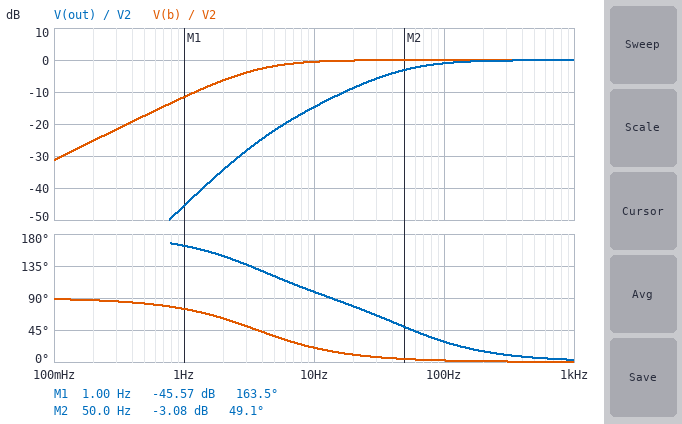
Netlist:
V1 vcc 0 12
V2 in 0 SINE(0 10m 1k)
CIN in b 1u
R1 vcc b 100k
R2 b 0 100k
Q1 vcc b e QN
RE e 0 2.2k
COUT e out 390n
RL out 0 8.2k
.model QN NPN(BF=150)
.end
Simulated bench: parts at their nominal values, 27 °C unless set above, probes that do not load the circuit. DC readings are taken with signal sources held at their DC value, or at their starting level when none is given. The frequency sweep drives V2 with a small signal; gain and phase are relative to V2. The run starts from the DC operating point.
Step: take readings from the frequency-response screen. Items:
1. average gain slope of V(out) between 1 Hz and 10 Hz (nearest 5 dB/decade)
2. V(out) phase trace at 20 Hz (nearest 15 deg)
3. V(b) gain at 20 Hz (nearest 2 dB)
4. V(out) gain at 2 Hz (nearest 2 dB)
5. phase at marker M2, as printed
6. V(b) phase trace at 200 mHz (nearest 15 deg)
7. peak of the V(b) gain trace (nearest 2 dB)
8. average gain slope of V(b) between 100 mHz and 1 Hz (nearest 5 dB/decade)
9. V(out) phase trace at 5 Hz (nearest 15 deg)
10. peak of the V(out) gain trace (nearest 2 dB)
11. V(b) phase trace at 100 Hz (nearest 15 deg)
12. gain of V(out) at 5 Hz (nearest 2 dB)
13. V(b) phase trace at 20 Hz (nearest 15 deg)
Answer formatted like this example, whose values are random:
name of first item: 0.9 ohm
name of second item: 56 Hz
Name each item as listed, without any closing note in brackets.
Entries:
average gain slope of V(out) between 1 Hz and 10 Hz: 30 dB/decade
V(out) phase trace at 20 Hz: 75 deg
V(b) gain at 20 Hz: 0 dB
V(out) gain at 2 Hz: -34 dB
phase at marker M2, as printed: 49.1 deg
V(b) phase trace at 200 mHz: 90 deg
peak of the V(b) gain trace: 0 dB
average gain slope of V(b) between 100 mHz and 1 Hz: 20 dB/decade
V(out) phase trace at 5 Hz: 120 deg
peak of the V(out) gain trace: 0 dB
V(b) phase trace at 100 Hz: 0 deg
gain of V(out) at 5 Hz: -22 dB
V(b) phase trace at 20 Hz: 15 deg
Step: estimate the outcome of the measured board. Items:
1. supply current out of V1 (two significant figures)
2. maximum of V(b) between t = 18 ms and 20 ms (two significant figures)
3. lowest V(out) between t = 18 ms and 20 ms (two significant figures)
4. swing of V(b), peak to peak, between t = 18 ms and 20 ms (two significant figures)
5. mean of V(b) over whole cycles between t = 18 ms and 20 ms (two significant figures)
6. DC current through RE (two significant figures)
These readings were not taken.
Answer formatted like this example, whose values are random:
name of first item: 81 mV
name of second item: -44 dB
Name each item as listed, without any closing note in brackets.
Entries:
supply current out of V1: 2.1 mA
maximum of V(b) between t = 18 ms and 20 ms: 5.3 V
lowest V(out) between t = 18 ms and 20 ms: -9.9 mV
swing of V(b), peak to peak, between t = 18 ms and 20 ms: 20 mV
mean of V(b) over whole cycles between t = 18 ms and 20 ms: 5.3 V
DC current through RE: 2.1 mA
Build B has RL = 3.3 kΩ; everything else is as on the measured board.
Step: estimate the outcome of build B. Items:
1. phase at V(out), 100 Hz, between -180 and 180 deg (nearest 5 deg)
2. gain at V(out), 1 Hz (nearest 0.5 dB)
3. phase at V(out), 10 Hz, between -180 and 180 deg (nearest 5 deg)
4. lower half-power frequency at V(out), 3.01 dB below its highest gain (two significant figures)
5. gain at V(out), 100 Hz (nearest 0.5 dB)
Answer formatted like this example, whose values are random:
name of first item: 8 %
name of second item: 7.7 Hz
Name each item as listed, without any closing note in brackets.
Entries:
phase at V(out), 100 Hz, between -180 and 180 deg: 55 deg
gain at V(out), 1 Hz: -53.5 dB
phase at V(out), 10 Hz, between -180 and 180 deg: 105 deg
lower half-power frequency at V(out), 3.01 dB below its highest gain: 120 Hz
gain at V(out), 100 Hz: -4.0 dB
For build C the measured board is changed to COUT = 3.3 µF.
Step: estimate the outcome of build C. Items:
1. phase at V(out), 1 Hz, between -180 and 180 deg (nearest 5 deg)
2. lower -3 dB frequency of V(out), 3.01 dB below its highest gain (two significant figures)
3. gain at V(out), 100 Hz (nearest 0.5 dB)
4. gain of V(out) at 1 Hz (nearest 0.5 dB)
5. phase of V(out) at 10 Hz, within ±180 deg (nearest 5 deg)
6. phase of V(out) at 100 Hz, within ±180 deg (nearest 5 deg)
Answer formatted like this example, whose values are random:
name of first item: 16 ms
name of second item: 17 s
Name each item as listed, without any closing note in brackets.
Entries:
phase at V(out), 1 Hz, between -180 and 180 deg: 155 deg
lower -3 dB frequency of V(out), 3.01 dB below its highest gain: 7.6 Hz
gain at V(out), 100 Hz: 0 dB
gain of V(out) at 1 Hz: -27.0 dB
phase of V(out) at 10 Hz, within ±180 deg: 50 deg
phase of V(out) at 100 Hz, within ±180 deg: 5 deg
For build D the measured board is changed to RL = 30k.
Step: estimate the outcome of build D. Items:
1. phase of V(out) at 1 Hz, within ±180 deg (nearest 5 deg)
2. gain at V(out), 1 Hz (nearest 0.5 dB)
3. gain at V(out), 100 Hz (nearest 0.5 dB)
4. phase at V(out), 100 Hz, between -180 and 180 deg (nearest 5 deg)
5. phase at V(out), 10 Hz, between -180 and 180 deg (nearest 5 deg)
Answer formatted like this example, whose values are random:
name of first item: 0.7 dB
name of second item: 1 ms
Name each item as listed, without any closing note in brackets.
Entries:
phase of V(out) at 1 Hz, within ±180 deg: 160 deg
gain at V(out), 1 Hz: -34.5 dB
gain at V(out), 100 Hz: 0 dB
phase at V(out), 100 Hz, between -180 and 180 deg: 10 deg
phase at V(out), 10 Hz, between -180 and 180 deg: 75 deg
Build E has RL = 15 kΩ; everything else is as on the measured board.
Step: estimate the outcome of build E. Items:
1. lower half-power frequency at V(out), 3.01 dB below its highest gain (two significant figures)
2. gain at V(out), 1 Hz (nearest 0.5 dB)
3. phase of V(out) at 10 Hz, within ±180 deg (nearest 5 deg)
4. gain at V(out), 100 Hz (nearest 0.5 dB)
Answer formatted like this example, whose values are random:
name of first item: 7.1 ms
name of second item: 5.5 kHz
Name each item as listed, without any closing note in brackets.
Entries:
lower half-power frequency at V(out), 3.01 dB below its highest gain: 28 Hz
gain at V(out), 1 Hz: -40.5 dB
phase of V(out) at 10 Hz, within ±180 deg: 90 deg
gain at V(out), 100 Hz: -0.5 dB
